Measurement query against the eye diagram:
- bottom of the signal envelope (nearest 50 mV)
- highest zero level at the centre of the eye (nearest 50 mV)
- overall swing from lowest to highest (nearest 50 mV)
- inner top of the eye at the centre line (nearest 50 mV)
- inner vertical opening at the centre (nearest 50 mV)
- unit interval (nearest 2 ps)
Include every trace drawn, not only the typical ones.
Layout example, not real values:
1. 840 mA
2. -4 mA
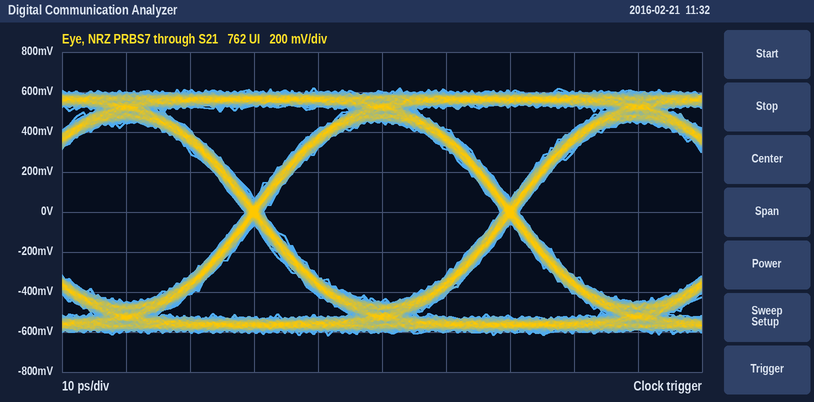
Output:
1. -600 mV
2. -450 mV
3. 1.25 V
4. 450 mV
5. 900 mV
6. 40 ps
